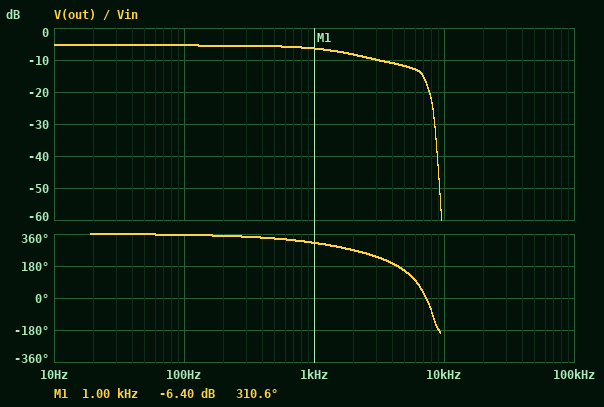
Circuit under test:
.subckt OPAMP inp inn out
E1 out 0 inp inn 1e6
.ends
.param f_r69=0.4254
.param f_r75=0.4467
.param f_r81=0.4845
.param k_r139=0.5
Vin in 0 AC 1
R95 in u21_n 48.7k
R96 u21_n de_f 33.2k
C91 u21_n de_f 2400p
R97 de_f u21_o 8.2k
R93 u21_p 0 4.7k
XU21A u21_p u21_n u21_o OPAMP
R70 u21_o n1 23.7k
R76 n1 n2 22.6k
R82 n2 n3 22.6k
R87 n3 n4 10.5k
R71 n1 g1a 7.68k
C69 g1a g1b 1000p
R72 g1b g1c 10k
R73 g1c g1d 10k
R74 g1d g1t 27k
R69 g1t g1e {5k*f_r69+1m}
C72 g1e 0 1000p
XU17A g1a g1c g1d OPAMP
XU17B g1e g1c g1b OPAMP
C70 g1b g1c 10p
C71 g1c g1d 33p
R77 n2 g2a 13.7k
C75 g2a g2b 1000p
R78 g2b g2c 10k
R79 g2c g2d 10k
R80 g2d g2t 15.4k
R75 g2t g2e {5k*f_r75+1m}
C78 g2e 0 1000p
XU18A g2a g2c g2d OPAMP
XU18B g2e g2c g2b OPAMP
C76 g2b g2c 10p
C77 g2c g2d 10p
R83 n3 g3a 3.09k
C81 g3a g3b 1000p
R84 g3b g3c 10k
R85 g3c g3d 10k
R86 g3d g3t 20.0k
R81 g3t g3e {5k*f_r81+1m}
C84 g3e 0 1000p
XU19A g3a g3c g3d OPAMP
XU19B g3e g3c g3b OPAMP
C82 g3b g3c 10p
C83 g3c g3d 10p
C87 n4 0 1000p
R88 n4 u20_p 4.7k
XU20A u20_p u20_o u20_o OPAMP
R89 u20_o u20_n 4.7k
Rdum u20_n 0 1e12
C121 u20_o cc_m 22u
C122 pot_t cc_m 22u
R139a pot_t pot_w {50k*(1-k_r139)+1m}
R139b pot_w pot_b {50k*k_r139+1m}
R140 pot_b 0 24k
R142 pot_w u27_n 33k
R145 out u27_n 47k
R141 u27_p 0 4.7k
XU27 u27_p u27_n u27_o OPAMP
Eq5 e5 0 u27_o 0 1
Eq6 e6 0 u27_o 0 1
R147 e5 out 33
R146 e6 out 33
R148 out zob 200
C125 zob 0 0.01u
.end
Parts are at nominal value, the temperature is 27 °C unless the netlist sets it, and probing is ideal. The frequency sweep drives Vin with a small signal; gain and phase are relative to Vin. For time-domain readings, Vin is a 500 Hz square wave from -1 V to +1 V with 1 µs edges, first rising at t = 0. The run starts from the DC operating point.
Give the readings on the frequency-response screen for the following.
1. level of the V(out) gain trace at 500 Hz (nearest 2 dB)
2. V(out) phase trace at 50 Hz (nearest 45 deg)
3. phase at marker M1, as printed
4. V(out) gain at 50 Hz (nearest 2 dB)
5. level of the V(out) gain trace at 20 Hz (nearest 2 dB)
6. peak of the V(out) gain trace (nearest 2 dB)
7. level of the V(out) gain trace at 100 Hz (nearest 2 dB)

-6 dB
360 deg
310.6 deg
-6 dB
-6 dB
-6 dB
-6 dB
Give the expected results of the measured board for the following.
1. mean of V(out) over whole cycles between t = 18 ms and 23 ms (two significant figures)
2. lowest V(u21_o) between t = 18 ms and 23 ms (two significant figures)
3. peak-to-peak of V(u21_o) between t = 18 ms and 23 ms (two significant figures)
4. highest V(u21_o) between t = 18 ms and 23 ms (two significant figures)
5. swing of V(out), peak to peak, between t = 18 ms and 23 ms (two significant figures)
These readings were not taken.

510 mV
-850 mV
1.7 V
850 mV
1.1 V
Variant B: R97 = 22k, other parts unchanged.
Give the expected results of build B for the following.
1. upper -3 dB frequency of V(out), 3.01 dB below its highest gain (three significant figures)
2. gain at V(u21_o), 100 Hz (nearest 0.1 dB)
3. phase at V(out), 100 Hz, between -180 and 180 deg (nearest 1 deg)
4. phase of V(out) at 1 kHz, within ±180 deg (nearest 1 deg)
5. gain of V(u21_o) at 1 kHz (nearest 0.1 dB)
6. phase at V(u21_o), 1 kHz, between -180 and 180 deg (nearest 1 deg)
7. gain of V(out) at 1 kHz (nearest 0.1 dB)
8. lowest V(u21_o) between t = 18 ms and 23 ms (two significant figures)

2.52 kHz
1.1 dB
-4 deg
-44 deg
0.3 dB
165 deg
-3.8 dB
-1.1 V
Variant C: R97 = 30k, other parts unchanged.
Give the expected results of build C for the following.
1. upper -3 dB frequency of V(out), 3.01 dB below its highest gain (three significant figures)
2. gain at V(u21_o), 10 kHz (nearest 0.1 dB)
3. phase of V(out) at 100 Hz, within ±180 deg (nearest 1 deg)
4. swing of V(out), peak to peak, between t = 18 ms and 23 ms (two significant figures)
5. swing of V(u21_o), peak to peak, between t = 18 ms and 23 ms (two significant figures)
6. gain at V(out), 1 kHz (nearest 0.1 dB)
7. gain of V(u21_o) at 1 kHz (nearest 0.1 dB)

2.99 kHz
-3.7 dB
-4 deg
1.7 V
2.6 V
-2.5 dB
1.5 dB
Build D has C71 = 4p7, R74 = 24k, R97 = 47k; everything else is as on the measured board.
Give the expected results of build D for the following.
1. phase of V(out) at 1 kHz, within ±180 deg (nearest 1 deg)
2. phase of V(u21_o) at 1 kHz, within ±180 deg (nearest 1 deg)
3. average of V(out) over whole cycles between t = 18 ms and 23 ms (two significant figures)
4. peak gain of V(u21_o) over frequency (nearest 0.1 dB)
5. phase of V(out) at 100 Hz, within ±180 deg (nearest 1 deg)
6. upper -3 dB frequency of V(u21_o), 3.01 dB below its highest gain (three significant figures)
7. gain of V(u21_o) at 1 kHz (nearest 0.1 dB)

-39 deg
170 deg
990 mV
4.3 dB
-4 deg
3.57 kHz
3.7 dB
